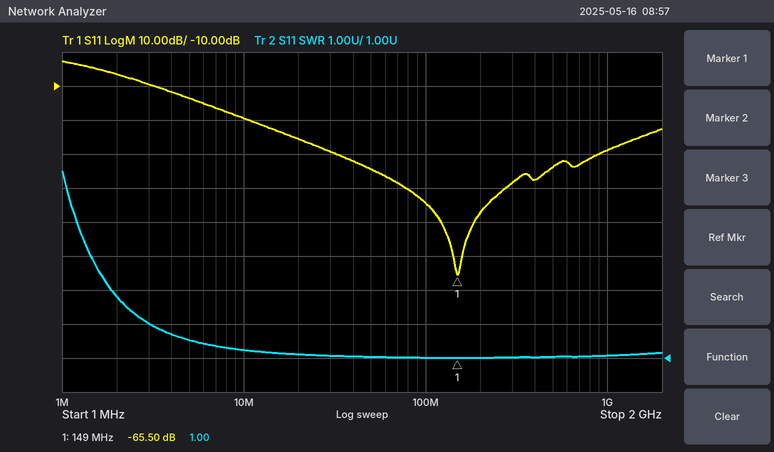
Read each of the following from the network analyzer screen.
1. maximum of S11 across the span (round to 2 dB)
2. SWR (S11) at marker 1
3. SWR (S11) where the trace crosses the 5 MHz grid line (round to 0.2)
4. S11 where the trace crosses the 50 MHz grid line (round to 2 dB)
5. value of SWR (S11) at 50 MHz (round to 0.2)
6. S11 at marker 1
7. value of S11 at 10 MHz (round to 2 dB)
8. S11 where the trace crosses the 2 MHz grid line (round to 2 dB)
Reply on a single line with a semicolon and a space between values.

-2 dB; 1.00; 1.6; -34 dB; 1.0; -65.50 dB; -20 dB; -6 dB
